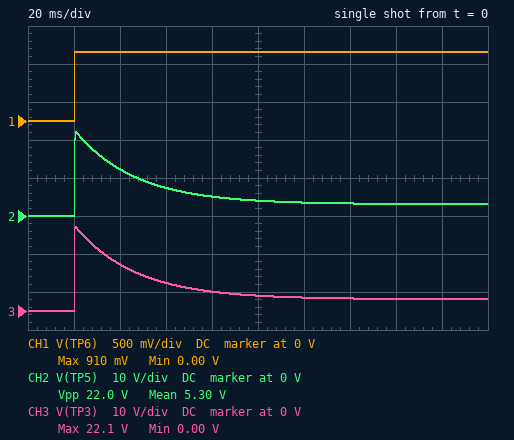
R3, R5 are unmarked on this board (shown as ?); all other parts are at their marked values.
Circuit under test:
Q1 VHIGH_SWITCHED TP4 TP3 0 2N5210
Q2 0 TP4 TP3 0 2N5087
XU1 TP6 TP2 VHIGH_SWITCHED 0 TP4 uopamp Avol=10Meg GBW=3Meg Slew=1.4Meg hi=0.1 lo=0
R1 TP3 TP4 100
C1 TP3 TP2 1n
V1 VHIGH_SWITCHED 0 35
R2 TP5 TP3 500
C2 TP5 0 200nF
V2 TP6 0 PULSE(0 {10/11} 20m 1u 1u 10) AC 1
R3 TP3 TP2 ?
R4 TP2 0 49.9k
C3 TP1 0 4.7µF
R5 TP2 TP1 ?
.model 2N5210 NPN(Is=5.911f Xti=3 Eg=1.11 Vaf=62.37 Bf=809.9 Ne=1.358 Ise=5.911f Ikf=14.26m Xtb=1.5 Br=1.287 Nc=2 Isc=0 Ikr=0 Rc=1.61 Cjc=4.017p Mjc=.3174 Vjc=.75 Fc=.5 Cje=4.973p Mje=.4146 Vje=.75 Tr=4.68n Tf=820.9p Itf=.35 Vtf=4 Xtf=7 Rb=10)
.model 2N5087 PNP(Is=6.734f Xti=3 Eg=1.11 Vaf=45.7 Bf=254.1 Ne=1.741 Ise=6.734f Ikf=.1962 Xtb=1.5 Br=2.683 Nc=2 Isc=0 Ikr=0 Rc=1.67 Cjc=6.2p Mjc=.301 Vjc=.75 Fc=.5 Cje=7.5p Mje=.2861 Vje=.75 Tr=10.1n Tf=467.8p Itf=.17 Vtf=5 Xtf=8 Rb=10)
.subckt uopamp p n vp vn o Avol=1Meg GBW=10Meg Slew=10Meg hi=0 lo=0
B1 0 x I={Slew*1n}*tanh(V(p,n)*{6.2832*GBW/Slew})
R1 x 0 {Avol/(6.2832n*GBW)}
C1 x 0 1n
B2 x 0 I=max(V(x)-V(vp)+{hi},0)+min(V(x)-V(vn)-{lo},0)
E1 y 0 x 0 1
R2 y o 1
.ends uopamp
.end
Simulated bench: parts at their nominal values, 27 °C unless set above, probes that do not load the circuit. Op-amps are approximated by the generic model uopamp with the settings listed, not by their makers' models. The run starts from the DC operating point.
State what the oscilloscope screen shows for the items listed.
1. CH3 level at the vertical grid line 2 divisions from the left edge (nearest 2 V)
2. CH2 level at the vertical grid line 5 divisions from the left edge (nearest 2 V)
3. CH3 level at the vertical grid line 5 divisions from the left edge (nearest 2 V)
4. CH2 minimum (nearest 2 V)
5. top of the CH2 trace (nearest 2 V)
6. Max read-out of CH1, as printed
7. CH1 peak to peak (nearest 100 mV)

12 V
4 V
4 V
0 V
22 V
910 mV
900 mV
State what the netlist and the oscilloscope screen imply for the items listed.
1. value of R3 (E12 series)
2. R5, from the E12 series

120 kΩ
5.6 kΩ
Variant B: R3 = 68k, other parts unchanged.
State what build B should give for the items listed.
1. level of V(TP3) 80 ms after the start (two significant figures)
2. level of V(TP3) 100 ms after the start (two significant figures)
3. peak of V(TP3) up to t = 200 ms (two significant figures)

3.3 V
2.7 V
13 V
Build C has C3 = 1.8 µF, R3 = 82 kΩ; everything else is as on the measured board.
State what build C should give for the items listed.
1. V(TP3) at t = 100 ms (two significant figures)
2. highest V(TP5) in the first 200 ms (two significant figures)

2.4 V
15 V
